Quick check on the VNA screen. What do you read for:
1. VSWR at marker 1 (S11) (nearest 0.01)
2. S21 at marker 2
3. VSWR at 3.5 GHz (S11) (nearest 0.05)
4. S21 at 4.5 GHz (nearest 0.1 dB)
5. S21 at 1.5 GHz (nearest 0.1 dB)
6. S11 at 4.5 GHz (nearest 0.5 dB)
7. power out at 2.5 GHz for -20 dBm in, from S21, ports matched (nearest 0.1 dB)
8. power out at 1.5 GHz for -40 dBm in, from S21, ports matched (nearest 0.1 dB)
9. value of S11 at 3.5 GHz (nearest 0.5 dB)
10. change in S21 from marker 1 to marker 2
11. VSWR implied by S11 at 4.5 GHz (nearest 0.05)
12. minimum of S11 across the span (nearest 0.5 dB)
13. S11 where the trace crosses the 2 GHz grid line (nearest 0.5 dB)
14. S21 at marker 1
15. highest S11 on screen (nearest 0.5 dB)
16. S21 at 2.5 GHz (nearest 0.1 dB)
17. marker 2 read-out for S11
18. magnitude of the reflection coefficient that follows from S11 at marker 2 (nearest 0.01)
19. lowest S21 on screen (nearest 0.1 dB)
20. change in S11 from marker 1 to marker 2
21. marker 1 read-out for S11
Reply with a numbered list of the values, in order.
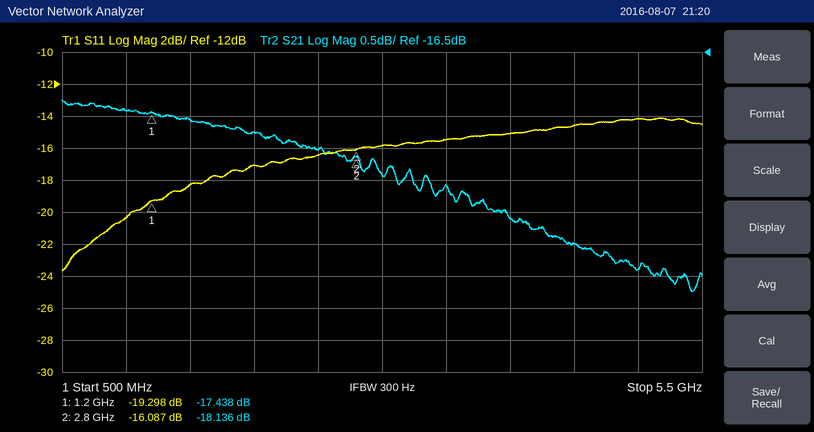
1. 1.24
2. -18.136 dB
3. 1.40
4. -19.5 dB
5. -17.6 dB
6. -14.5 dB
7. -38.0 dBm
8. -57.6 dBm
9. -15.5 dB
10. -0.698 dB
11. 1.45
12. -23.5 dB
13. -17.0 dB
14. -17.438 dB
15. -14.0 dB
16. -18.0 dB
17. -16.087 dB
18. 0.16
19. -20.2 dB
20. 3.211 dB
21. -19.298 dB
